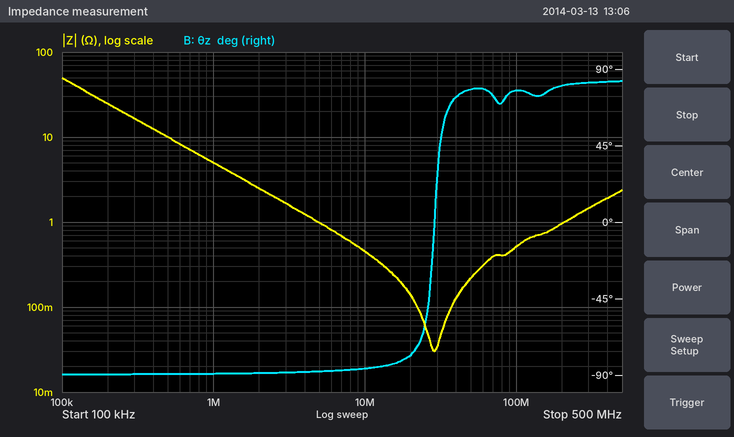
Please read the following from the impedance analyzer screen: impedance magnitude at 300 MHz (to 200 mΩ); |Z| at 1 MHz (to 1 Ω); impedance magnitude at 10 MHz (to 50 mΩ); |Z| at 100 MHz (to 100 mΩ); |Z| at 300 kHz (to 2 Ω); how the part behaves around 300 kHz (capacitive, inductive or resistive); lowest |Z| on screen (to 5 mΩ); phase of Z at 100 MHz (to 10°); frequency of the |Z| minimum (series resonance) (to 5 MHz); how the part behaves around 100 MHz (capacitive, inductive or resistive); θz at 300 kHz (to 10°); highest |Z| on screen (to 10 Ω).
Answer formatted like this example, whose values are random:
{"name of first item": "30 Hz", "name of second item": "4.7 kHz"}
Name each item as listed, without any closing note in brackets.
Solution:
{"impedance magnitude at 300 MHz": "1.4 Ω", "|Z| at 1 MHz": "5 Ω", "impedance magnitude at 10 MHz": "450 mΩ", "|Z| at 100 MHz": "500 mΩ", "|Z| at 300 kHz": "16 Ω", "how the part behaves around 300 kHz": "capacitive", "lowest |Z| on screen": "30 mΩ", "phase of Z at 100 MHz": "80°", "frequency of the |Z| minimum (series resonance)": "30 MHz", "how the part behaves around 100 MHz": "inductive", "θz at 300 kHz": "-90°", "highest |Z| on screen": "50 Ω"}
